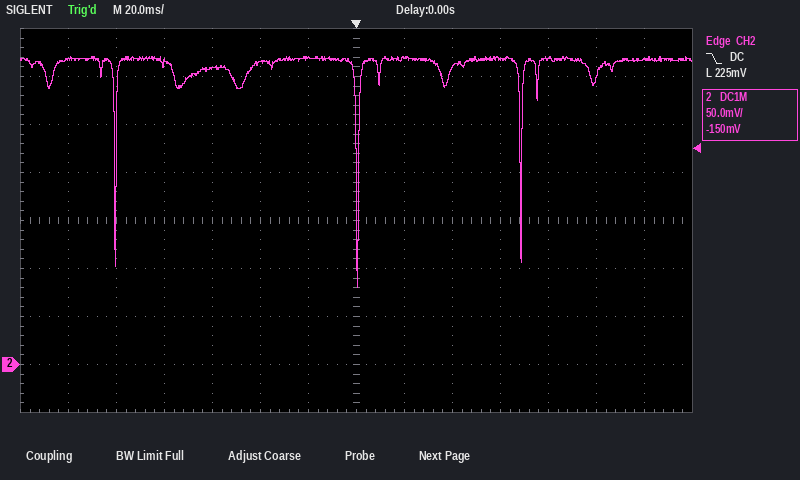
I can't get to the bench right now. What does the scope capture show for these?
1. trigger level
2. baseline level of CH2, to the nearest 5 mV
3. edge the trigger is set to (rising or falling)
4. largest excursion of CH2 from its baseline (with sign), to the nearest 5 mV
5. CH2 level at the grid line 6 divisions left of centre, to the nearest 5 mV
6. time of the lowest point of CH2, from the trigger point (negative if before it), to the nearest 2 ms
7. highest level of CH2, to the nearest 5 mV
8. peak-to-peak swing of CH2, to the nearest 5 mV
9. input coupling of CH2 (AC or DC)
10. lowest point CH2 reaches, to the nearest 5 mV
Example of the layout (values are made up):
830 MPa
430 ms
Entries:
225 mV
320 mV
falling
-240 mV
320 mV
0 ms
320 mV
240 mV
DC
80 mV
